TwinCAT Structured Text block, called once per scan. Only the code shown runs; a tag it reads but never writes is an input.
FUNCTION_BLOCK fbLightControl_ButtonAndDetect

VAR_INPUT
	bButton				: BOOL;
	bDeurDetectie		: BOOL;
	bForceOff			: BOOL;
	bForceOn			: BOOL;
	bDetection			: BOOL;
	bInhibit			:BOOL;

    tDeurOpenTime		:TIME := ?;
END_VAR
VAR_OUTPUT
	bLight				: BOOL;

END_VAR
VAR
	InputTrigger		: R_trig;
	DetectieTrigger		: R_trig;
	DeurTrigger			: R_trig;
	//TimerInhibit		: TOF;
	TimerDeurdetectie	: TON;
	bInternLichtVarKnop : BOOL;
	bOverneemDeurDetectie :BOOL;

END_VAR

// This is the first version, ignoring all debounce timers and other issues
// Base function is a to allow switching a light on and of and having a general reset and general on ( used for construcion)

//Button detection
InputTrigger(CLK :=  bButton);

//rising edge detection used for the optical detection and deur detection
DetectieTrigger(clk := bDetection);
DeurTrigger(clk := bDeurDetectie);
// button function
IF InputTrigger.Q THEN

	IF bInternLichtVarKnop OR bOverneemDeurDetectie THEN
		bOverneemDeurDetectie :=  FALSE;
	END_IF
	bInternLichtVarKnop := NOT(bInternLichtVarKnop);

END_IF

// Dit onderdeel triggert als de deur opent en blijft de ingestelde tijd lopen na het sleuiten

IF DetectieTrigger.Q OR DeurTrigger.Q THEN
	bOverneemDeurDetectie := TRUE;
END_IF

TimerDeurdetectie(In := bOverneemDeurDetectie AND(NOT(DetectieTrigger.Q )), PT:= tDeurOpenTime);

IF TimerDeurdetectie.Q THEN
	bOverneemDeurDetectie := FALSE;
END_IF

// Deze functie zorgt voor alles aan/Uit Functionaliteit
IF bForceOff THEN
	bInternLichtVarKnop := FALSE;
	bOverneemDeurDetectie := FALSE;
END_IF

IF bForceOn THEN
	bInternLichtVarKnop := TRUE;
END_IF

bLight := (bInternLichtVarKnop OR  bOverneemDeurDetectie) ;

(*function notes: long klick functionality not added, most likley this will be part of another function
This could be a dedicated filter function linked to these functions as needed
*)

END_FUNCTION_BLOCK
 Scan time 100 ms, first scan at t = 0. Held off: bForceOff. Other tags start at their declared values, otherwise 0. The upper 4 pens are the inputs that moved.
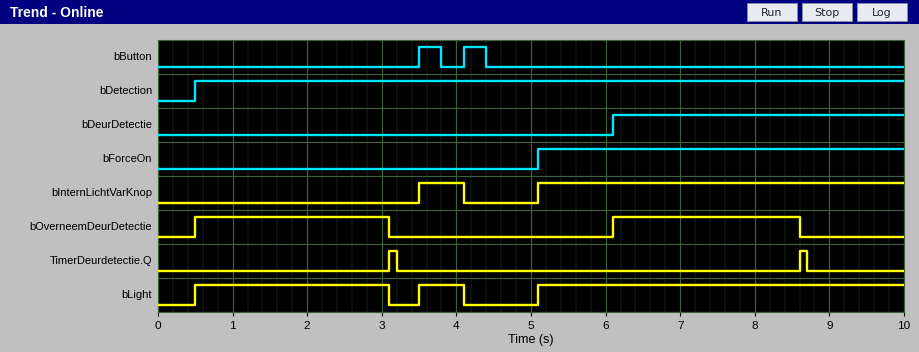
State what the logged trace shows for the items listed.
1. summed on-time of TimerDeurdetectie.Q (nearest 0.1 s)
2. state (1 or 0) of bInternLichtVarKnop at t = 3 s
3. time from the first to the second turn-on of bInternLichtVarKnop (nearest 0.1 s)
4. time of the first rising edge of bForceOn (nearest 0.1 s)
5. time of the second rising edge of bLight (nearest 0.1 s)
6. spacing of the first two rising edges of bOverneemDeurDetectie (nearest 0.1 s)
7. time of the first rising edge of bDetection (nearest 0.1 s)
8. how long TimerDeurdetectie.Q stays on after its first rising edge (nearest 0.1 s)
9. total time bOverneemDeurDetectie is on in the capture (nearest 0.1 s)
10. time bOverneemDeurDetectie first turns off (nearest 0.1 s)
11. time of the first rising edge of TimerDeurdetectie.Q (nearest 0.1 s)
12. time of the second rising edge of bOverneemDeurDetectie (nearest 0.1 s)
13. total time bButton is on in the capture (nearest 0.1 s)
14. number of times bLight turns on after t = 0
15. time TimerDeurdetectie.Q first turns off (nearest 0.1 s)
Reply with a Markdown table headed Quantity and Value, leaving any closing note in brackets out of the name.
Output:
| Quantity | Value |
|---|---|
| summed on-time of TimerDeurdetectie.Q | 0.2 s |
| state (1 or 0) of bInternLichtVarKnop at t = 3 s | 0 |
| time from the first to the second turn-on of bInternLichtVarKnop | 1.6 s |
| time of the first rising edge of bForceOn | 5.1 s |
| time of the second rising edge of bLight | 3.5 s |
| spacing of the first two rising edges of bOverneemDeurDetectie | 5.6 s |
| time of the first rising edge of bDetection | 0.5 s |
| how long TimerDeurdetectie.Q stays on after its first rising edge | 0.1 s |
| total time bOverneemDeurDetectie is on in the capture | 5.1 s |
| time bOverneemDeurDetectie first turns off | 3.1 s |
| time of the first rising edge of TimerDeurdetectie.Q | 3.1 s |
| time of the second rising edge of bOverneemDeurDetectie | 6.1 s |
| total time bButton is on in the capture | 0.6 s |
| number of times bLight turns on after t = 0 | 3 |
| time TimerDeurdetectie.Q first turns off | 3.2 s |
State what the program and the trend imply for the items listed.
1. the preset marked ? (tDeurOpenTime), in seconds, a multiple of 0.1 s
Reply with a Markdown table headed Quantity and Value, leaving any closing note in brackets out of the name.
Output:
| Quantity | Value |
|---|---|
| the preset marked ? (tDeurOpenTime), in seconds, a multiple of 0.1 s | 2.5 s |
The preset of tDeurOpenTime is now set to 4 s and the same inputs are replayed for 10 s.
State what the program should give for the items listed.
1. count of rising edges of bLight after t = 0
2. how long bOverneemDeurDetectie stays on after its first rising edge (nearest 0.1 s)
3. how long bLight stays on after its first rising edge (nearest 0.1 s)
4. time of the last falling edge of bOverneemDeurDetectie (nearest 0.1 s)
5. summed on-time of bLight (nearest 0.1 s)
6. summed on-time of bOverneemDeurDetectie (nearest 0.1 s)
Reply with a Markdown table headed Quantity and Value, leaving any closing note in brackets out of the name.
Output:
| Quantity | Value |
|---|---|
| count of rising edges of bLight after t = 0 | 2 |
| how long bOverneemDeurDetectie stays on after its first rising edge | 3.0 s |
| how long bLight stays on after its first rising edge | 3.6 s |
| time of the last falling edge of bOverneemDeurDetectie | 3.5 s |
| summed on-time of bLight | 8.5 s |
| summed on-time of bOverneemDeurDetectie | 6.9 s |
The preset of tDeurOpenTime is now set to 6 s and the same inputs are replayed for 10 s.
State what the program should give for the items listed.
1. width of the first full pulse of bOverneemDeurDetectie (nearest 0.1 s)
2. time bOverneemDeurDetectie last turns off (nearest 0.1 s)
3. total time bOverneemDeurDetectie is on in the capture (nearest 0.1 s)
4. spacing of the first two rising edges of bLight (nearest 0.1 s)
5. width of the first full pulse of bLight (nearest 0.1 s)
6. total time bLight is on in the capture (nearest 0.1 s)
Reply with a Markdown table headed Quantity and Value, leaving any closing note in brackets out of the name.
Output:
| Quantity | Value |
|---|---|
| width of the first full pulse of bOverneemDeurDetectie | 3.0 s |
| time bOverneemDeurDetectie last turns off | 3.5 s |
| total time bOverneemDeurDetectie is on in the capture | 6.9 s |
| spacing of the first two rising edges of bLight | 4.6 s |
| width of the first full pulse of bLight | 3.6 s |
| total time bLight is on in the capture | 8.5 s |
